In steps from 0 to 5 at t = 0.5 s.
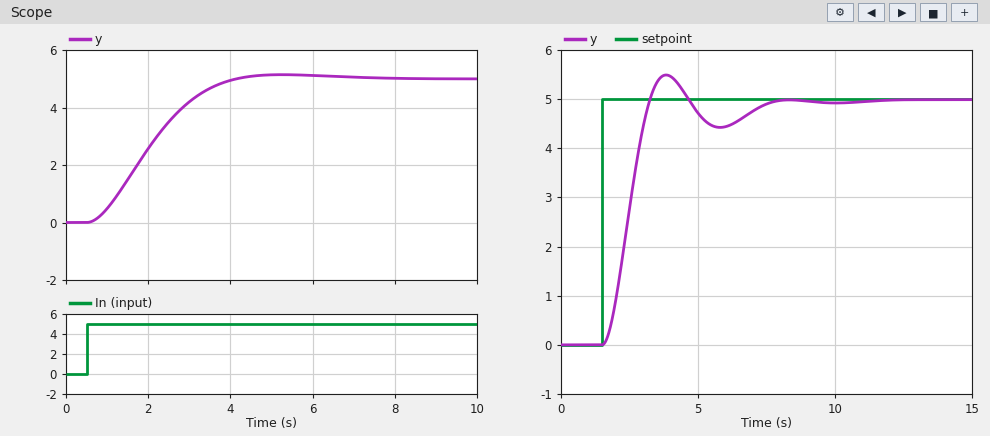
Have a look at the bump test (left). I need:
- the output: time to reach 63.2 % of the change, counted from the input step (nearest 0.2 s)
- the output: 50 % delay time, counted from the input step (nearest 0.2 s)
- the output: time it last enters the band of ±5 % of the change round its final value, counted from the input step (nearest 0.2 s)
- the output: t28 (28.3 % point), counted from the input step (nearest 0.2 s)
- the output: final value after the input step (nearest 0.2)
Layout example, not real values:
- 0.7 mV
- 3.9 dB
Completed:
- 1.8 s
- 1.4 s
- 3.2 s
- 1.0 s
- 5.0
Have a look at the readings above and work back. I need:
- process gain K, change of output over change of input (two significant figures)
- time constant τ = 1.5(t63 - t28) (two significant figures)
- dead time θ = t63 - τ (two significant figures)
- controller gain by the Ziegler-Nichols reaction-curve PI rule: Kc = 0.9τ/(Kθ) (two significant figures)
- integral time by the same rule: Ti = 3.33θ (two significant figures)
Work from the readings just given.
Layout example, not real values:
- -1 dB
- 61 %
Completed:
- 1.0
- 1.2 s
- 0.60 s
- 1.8
- 2.0 s
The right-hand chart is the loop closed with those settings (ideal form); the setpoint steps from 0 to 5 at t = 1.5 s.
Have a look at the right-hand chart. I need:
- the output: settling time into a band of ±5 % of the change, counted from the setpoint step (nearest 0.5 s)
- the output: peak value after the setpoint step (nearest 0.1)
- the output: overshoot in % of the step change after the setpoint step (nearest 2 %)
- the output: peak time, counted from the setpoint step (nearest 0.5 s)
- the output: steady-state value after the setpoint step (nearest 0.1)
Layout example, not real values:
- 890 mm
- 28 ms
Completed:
- 5.5 s
- 5.5
- 10 %
- 2.5 s
- 5.0
